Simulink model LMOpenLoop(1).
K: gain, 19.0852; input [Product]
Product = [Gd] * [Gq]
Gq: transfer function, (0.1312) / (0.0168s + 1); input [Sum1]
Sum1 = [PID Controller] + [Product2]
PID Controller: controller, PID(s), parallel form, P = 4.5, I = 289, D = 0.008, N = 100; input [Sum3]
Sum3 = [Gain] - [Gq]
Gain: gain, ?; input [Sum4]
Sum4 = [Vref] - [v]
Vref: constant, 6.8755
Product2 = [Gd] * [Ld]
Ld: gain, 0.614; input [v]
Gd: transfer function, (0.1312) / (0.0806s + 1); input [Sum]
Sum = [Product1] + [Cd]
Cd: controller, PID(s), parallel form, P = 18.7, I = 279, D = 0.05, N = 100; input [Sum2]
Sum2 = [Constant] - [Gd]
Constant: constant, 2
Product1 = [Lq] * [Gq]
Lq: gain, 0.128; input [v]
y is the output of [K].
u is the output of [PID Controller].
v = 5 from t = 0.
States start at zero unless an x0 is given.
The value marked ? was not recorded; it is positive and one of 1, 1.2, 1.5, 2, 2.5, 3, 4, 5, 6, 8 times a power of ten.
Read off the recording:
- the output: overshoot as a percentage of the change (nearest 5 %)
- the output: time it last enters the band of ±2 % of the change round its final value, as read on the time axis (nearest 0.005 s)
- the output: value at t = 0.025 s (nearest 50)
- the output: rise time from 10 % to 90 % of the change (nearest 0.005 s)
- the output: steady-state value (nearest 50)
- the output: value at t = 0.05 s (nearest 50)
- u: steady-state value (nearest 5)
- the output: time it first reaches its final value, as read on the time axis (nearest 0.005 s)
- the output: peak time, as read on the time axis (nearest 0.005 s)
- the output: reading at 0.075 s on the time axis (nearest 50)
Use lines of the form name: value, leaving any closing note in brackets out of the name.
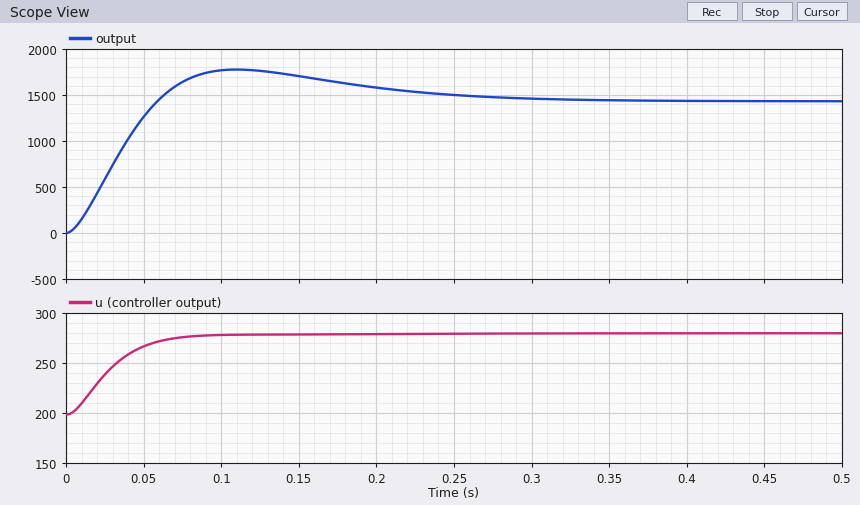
the output: overshoot as a percentage of the change: 25 %
the output: time it last enters the band of ±2 % of the change round its final value, as read on the time axis: 0.300 s
the output: value at t = 0.025 s: 600
the output: rise time from 10 % to 90 % of the change: 0.040 s
the output: steady-state value: 1450
the output: value at t = 0.05 s: 1250
u: steady-state value: 280
the output: time it first reaches its final value, as read on the time axis: 0.060 s
the output: peak time, as read on the time axis: 0.110 s
the output: reading at 0.075 s on the time axis: 1650
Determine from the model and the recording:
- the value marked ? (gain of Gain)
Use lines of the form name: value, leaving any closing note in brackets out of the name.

the value marked ?: 20
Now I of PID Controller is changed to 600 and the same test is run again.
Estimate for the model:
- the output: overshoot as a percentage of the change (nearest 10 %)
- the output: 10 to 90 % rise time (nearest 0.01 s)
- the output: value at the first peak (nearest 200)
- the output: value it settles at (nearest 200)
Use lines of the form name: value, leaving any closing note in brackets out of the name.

the output: overshoot as a percentage of the change: 30 %
the output: 10 to 90 % rise time: 0.03 s
the output: value at the first peak: 1800
the output: value it settles at: 1400
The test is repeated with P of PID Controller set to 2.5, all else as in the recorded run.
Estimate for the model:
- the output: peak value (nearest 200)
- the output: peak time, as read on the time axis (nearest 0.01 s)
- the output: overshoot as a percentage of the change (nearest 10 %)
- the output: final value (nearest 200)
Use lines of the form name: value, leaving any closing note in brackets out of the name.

the output: peak value: 1800
the output: peak time, as read on the time axis: 0.10 s
the output: overshoot as a percentage of the change: 30 %
the output: final value: 1400
